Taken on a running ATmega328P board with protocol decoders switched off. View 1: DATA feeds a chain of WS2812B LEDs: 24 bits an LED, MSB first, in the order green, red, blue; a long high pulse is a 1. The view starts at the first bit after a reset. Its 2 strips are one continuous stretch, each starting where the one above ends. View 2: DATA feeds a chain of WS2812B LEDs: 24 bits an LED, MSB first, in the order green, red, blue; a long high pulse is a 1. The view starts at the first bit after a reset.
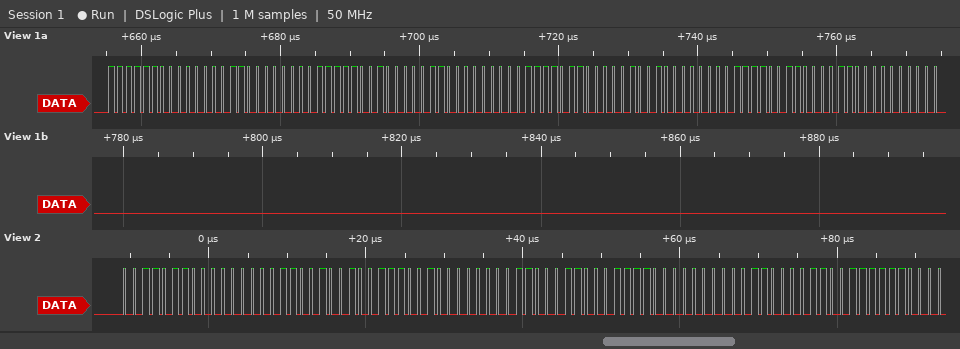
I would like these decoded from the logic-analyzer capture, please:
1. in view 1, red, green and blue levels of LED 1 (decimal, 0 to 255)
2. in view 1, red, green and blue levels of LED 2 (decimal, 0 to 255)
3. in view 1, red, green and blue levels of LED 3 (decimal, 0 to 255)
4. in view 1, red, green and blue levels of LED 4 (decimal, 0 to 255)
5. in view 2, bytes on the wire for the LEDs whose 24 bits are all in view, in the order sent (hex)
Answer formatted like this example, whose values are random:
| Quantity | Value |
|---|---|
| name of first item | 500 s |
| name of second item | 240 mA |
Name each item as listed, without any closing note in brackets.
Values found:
| Quantity | Value |
|---|---|
| in view 1, red, green and blue levels of LED 1 | 3, 252, 0 |
| in view 1, red, green and blue levels of LED 2 | 6, 249, 0 |
| in view 1, red, green and blue levels of LED 3 | 9, 246, 0 |
| in view 1, red, green and blue levels of LED 4 | 12, 243, 0 |
| in view 2, bytes on the wire for the LEDs whose 24 bits are all in view, in the order sent | 36 00 C9 39 00 C6 3C 00 C3 |
